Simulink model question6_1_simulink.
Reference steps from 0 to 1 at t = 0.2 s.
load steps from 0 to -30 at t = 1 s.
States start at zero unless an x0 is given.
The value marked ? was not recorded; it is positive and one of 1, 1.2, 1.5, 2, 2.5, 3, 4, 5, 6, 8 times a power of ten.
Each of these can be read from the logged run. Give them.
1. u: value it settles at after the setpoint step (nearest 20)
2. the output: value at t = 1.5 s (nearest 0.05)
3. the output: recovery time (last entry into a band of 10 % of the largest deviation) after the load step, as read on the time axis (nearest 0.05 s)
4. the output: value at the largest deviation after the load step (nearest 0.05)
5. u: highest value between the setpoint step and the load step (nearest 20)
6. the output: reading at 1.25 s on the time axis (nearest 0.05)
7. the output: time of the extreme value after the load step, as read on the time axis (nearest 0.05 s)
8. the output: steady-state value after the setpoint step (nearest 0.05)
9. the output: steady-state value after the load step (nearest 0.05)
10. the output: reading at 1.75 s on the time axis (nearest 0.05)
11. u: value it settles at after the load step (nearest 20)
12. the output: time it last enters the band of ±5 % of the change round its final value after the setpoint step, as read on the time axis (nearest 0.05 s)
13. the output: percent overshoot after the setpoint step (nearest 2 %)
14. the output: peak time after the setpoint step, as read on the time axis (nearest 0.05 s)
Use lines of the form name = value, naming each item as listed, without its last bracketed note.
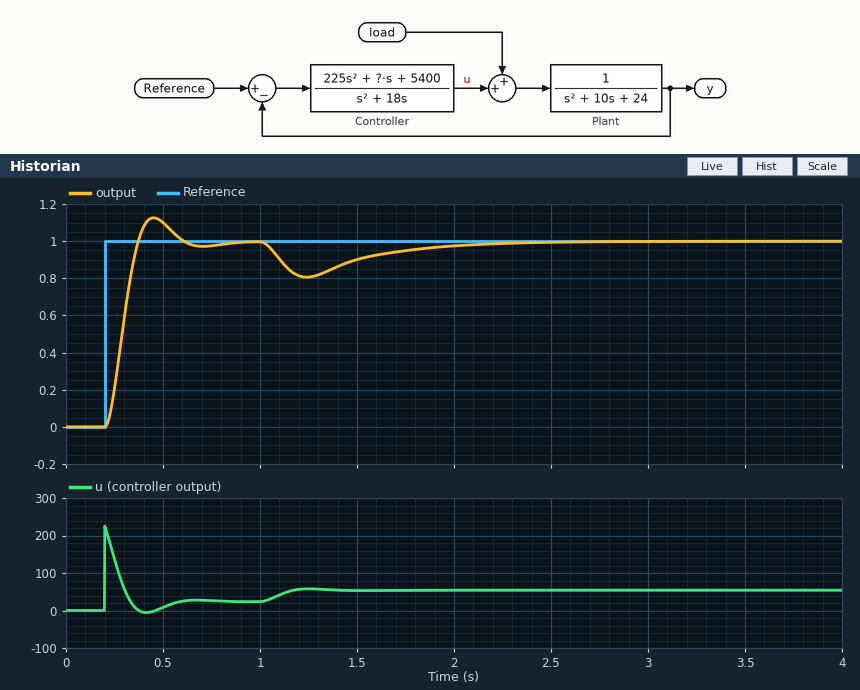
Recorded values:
u: value it settles at after the setpoint step = 20
the output: value at t = 1.5 s = 0.90
the output: recovery time (last entry into a band of 10 % of the largest deviation) after the load step, as read on the time axis = 2.10 s
the output: value at the largest deviation after the load step = 0.80
u: highest value between the setpoint step and the load step = 220
the output: reading at 1.25 s on the time axis = 0.80
the output: time of the extreme value after the load step, as read on the time axis = 1.25 s
the output: steady-state value after the setpoint step = 1.00
the output: steady-state value after the load step = 1.00
the output: reading at 1.75 s on the time axis = 0.95
u: value it settles at after the load step = 60
the output: time it last enters the band of ±5 % of the change round its final value after the setpoint step, as read on the time axis = 0.55 s
the output: percent overshoot after the setpoint step = 12 %
the output: peak time after the setpoint step, as read on the time axis = 0.45 s
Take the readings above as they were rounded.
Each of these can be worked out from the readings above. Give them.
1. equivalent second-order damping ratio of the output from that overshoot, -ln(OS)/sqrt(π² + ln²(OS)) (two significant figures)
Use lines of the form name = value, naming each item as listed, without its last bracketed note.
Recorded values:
equivalent second-order damping ratio of the output from that overshoot, -ln(OS)/sqrt(π² + ln²(OS)) = 0.56
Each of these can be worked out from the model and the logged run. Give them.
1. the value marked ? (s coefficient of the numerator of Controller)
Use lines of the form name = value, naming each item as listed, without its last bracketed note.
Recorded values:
the value marked ? = 2500
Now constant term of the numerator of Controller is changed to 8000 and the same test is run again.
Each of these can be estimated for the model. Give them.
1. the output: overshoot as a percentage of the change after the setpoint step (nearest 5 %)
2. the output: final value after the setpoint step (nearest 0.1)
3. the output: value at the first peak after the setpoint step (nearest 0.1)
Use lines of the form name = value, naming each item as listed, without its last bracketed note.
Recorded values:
the output: overshoot as a percentage of the change after the setpoint step = 20 %
the output: final value after the setpoint step = 1.0
the output: value at the first peak after the setpoint step = 1.2
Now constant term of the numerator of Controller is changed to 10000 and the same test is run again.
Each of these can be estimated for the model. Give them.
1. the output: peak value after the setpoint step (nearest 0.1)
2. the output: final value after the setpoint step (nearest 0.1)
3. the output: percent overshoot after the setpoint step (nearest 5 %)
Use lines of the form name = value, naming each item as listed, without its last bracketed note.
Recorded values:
the output: peak value after the setpoint step = 1.2
the output: final value after the setpoint step = 1.0
the output: percent overshoot after the setpoint step = 25 %
